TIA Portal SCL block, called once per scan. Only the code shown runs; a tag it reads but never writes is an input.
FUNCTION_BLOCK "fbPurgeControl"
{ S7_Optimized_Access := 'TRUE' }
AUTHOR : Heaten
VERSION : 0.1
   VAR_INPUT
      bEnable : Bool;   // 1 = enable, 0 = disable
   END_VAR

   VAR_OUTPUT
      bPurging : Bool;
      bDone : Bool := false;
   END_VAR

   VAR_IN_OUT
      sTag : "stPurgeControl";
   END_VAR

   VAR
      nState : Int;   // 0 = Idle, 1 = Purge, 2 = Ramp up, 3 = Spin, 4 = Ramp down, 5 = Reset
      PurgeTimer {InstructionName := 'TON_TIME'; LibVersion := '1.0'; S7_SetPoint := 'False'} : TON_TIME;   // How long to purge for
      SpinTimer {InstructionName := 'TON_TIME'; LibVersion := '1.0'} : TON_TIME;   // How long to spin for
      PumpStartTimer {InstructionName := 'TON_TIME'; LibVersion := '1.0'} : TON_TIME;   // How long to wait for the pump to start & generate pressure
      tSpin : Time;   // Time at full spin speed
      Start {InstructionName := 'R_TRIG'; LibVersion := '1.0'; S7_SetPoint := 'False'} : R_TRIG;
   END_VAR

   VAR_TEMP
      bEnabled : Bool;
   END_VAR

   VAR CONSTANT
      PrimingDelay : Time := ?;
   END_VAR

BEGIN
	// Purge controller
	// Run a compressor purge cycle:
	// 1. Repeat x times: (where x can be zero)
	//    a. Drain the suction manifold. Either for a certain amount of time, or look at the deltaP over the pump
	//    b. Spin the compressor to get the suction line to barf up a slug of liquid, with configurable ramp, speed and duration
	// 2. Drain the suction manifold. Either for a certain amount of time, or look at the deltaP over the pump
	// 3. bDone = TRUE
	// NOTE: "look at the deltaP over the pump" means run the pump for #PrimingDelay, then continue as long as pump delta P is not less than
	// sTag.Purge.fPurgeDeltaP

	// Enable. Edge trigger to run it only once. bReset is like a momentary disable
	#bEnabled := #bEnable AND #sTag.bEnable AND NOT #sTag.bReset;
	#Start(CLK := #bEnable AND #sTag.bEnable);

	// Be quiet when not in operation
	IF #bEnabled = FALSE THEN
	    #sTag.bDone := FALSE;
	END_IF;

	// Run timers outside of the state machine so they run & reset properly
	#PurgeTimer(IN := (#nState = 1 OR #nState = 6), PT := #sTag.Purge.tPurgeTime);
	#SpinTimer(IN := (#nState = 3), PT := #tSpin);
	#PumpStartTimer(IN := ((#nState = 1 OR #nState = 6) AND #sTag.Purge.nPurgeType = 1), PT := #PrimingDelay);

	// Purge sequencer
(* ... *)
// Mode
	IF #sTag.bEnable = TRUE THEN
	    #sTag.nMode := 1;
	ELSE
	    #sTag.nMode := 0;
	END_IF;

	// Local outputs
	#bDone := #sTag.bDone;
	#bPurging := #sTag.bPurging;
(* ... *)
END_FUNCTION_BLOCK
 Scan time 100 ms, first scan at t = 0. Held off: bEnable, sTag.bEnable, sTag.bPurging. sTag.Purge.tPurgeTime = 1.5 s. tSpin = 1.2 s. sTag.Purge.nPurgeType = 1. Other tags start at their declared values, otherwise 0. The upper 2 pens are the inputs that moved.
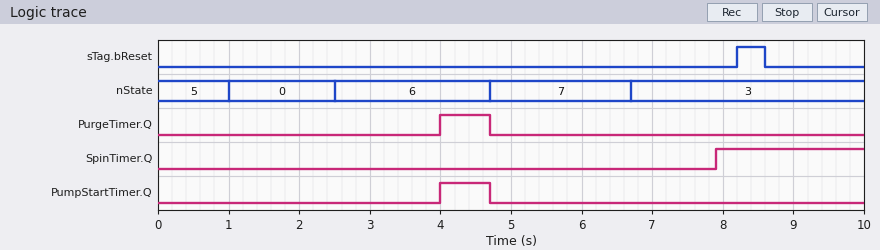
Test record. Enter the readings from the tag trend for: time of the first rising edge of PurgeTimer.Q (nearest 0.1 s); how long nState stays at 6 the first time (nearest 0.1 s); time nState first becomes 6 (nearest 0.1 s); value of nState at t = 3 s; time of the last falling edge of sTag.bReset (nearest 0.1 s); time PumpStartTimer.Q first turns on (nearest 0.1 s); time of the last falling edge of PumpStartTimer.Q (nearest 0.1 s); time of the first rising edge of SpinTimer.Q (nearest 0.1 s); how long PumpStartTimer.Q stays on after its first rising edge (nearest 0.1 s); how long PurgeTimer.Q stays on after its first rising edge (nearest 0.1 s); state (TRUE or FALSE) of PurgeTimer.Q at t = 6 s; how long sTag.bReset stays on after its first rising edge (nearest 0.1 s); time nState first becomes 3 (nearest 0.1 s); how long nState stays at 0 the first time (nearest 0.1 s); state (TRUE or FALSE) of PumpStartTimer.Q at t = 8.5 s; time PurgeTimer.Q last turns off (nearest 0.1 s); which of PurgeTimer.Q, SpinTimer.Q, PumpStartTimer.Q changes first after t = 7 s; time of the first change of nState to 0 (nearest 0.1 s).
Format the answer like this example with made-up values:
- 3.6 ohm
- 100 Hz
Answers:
- 4.0 s
- 2.2 s
- 2.5 s
- 6
- 8.6 s
- 4.0 s
- 4.7 s
- 7.9 s
- 0.7 s
- 0.7 s
- FALSE
- 0.4 s
- 6.7 s
- 1.5 s
- FALSE
- 4.7 s
- SpinTimer.Q
- 1.0 s
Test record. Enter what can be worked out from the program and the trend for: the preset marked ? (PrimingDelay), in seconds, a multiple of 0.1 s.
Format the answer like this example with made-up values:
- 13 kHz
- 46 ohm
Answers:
- 1.5 s
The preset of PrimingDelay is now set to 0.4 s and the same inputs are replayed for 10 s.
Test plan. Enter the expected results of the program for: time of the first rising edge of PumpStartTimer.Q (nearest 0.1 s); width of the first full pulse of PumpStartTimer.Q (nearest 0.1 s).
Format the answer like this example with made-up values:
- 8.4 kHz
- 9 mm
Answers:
- 2.9 s
- 1.8 s
